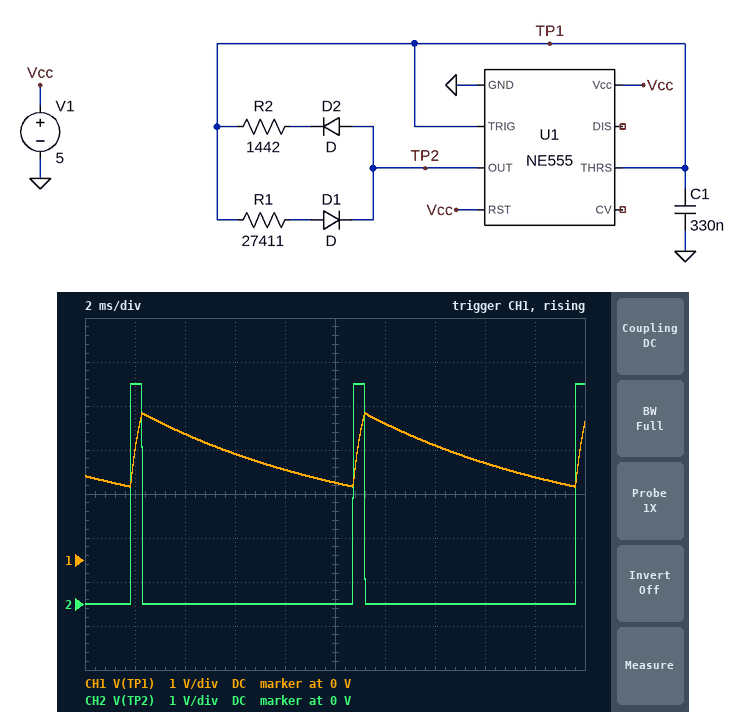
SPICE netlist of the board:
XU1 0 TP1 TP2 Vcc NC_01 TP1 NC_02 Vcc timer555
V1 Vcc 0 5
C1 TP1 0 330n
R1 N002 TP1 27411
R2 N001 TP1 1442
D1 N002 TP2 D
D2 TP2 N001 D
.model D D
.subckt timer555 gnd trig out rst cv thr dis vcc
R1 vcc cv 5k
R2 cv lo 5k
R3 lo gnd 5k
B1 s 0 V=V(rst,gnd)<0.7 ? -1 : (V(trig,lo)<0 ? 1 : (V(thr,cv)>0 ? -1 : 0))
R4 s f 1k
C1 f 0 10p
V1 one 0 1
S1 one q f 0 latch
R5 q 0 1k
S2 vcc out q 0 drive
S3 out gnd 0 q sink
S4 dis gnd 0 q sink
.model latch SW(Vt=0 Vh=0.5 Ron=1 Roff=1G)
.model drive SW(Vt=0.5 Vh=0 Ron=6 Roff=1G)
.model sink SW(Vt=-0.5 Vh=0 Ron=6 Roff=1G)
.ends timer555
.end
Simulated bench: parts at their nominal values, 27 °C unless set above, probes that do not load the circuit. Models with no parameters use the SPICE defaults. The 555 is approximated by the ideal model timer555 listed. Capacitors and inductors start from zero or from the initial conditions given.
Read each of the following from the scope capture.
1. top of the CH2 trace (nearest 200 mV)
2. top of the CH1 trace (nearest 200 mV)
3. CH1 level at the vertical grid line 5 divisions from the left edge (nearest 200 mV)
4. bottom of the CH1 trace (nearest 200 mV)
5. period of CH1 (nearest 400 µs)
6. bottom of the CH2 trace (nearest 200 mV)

5.0 V
3.4 V
1.8 V
1.6 V
8.8 ms
0 V
